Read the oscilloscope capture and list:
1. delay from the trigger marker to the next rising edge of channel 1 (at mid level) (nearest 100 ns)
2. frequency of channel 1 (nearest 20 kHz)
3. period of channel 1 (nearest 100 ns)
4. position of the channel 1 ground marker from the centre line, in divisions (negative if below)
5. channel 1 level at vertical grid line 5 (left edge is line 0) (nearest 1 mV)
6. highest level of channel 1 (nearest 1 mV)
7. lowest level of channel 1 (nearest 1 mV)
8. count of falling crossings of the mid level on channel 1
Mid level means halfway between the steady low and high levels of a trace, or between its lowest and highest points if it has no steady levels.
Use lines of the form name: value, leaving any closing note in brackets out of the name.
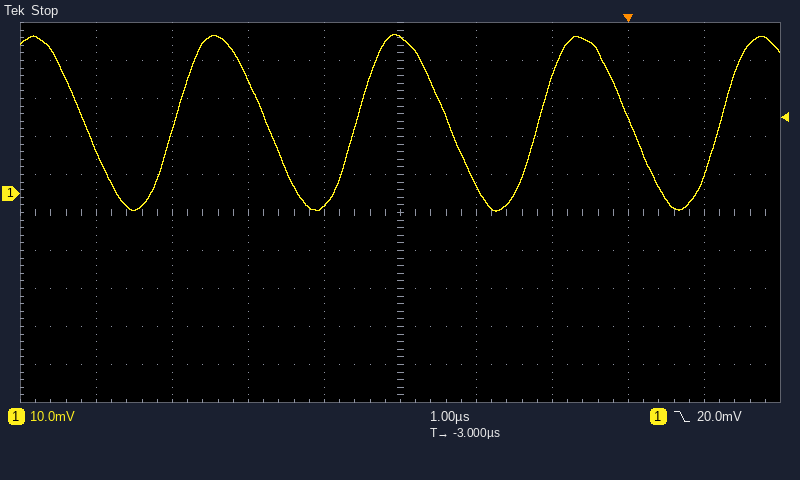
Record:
delay from the trigger marker to the next rising edge of channel 1 (at mid level): 1.2 µs
frequency of channel 1: 420 kHz
period of channel 1: 2.4 µs
position of the channel 1 ground marker from the centre line, in divisions: +0.5 div
channel 1 level at vertical grid line 5 (left edge is line 0): 41 mV
highest level of channel 1: 42 mV
lowest level of channel 1: -5 mV
count of falling crossings of the mid level on channel 1: 4
